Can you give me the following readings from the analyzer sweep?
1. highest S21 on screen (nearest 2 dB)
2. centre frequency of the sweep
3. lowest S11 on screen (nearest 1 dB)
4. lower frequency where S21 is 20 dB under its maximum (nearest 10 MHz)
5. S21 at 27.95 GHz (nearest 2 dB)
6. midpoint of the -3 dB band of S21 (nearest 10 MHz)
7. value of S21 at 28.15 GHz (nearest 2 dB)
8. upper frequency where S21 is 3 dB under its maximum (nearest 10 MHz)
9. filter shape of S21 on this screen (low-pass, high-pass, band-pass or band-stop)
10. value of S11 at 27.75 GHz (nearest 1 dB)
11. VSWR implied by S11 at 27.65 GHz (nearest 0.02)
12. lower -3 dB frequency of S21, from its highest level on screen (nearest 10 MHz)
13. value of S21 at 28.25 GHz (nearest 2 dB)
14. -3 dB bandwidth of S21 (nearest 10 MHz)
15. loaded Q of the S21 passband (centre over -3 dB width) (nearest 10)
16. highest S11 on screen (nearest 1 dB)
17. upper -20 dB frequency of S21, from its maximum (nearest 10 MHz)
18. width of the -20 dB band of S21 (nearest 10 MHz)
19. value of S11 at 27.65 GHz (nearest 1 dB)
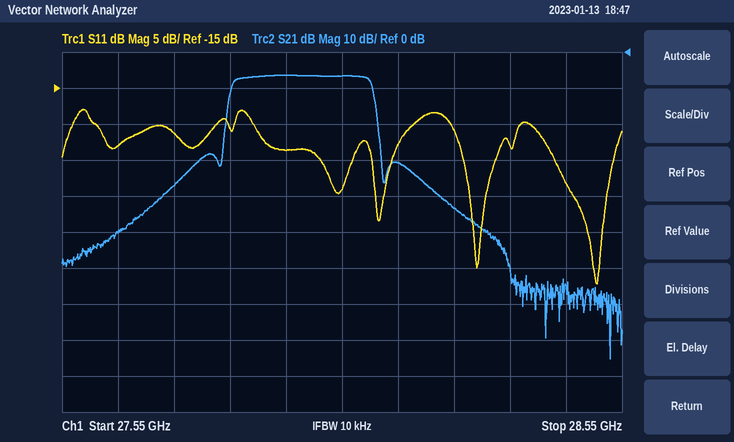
-6 dB
28.05 GHz
-42 dB
27.84 GHz
-6 dB
27.98 GHz
-30 dB
28.10 GHz
band-pass
-21 dB
1.16
27.85 GHz
-44 dB
250 MHz
110
-18 dB
28.12 GHz
280 MHz
-23 dB
